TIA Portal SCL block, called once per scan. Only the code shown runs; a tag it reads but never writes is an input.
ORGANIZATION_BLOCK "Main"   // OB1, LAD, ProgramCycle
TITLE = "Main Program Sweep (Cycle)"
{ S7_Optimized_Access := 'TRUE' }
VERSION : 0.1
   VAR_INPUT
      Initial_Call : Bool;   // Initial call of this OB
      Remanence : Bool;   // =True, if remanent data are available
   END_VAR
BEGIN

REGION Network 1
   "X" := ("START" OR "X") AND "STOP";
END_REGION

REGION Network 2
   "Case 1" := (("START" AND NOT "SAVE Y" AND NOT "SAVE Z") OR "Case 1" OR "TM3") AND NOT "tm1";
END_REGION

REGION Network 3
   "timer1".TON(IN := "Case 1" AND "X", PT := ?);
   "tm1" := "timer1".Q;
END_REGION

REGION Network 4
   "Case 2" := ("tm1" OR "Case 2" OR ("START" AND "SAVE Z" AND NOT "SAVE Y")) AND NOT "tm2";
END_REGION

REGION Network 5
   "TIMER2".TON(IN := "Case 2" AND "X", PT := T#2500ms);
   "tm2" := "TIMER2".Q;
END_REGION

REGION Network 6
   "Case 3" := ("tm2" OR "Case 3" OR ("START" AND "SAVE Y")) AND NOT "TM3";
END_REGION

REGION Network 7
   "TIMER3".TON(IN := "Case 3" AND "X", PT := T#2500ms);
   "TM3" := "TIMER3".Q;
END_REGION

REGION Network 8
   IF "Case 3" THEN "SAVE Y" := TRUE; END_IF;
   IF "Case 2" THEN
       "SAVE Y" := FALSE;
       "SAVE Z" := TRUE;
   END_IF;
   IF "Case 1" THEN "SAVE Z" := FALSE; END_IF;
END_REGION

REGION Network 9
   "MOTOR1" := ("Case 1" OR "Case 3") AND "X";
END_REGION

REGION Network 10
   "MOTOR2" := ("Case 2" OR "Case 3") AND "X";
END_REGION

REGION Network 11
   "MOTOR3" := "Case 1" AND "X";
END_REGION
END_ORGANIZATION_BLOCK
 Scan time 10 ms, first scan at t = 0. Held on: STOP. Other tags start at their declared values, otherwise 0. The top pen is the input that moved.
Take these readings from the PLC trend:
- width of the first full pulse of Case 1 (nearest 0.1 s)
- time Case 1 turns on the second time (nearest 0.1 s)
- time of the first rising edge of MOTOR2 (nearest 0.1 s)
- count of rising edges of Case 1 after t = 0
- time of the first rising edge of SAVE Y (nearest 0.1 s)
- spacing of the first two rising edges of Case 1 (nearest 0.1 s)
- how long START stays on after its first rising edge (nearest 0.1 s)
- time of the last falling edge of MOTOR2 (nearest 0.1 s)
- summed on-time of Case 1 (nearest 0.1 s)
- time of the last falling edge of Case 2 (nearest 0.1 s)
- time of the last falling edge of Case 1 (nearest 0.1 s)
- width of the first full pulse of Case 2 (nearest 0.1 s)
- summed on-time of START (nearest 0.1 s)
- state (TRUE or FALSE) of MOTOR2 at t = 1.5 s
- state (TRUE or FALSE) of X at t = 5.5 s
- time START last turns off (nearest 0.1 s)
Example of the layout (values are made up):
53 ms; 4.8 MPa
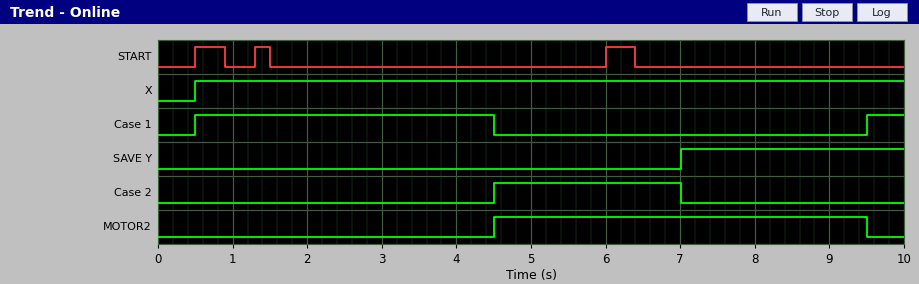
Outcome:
4.0 s; 9.5 s; 4.5 s; 2; 7.0 s; 9.0 s; 0.4 s; 9.5 s; 4.5 s; 7.0 s; 4.5 s; 2.5 s; 1.0 s; FALSE; TRUE; 6.4 s
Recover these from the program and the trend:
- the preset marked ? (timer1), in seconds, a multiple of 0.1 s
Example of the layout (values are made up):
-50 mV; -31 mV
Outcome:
4.0 s
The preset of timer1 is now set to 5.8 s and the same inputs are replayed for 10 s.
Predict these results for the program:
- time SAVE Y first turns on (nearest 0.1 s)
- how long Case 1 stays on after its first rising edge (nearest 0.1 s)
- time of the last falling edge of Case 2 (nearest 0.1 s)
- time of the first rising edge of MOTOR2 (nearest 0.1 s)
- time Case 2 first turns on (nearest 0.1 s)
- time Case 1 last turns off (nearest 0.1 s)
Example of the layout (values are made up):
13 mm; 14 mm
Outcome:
8.8 s; 5.8 s; 8.8 s; 6.3 s; 6.3 s; 6.3 s
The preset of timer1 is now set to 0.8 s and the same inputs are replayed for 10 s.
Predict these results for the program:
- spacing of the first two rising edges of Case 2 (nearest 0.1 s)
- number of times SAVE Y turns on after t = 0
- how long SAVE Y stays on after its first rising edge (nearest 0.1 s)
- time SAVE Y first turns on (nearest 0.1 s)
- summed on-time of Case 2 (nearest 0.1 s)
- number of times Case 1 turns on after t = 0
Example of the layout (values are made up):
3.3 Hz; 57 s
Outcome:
5.8 s; 2; 3.3 s; 3.8 s; 5.4 s; 3
